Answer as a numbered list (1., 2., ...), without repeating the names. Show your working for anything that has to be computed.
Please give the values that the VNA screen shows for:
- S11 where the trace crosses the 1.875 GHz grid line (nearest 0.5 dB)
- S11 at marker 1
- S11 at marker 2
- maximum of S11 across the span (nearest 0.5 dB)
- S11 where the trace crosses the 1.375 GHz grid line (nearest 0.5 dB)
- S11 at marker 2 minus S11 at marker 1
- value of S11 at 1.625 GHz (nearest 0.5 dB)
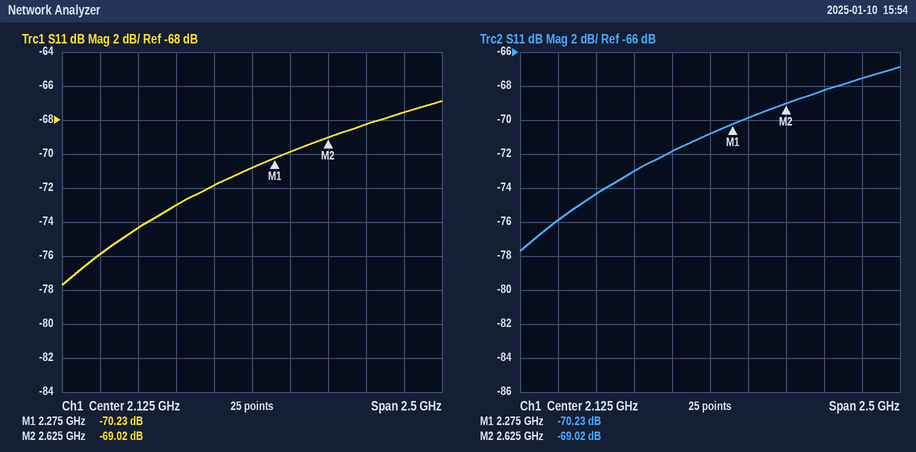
1. -72.0 dB
2. -70.23 dB
3. -69.02 dB
4. -67.0 dB
5. -74.5 dB
6. -69.02 − (-70.23) = 1.21 dB
7. -73.0 dB
